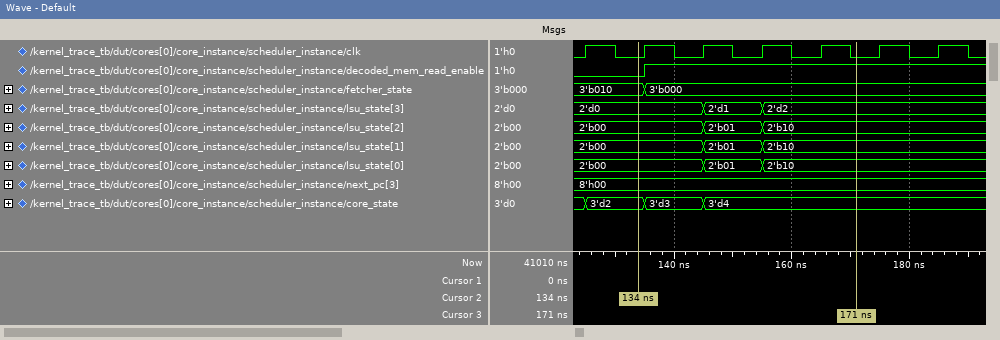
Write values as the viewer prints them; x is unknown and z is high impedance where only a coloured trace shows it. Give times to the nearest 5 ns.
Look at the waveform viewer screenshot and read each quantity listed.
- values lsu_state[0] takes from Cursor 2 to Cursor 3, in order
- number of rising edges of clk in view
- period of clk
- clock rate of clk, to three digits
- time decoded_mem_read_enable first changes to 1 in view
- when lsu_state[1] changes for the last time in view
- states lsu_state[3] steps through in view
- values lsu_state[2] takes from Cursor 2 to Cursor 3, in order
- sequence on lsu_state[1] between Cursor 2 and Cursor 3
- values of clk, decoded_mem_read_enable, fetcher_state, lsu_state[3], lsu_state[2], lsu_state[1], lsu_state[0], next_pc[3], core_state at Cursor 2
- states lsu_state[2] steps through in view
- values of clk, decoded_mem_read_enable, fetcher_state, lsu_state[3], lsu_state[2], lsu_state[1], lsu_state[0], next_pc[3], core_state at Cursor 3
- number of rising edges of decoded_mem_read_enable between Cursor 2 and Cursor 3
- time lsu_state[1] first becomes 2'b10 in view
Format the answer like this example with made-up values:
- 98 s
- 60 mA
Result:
- 2'b00, 2'b01, 2'b10
- 7
- 10 ns
- 100 MHz
- 135 ns
- 155 ns
- 2'd0, 2'd1, 2'd2
- 2'b00, 2'b01, 2'b10
- 2'b00, 2'b01, 2'b10
- clk=0, decoded_mem_read_enable=0, fetcher_state=3'b010, lsu_state[3]=2'd0, lsu_state[2]=2'b00, lsu_state[1]=2'b00, lsu_state[0]=2'b00, next_pc[3]=8'h00, core_state=3'd2
- 2'b00, 2'b01, 2'b10
- clk=0, decoded_mem_read_enable=1, fetcher_state=3'b000, lsu_state[3]=2'd2, lsu_state[2]=2'b10, lsu_state[1]=2'b10, lsu_state[0]=2'b10, next_pc[3]=8'h00, core_state=3'd4
- 1
- 155 ns
